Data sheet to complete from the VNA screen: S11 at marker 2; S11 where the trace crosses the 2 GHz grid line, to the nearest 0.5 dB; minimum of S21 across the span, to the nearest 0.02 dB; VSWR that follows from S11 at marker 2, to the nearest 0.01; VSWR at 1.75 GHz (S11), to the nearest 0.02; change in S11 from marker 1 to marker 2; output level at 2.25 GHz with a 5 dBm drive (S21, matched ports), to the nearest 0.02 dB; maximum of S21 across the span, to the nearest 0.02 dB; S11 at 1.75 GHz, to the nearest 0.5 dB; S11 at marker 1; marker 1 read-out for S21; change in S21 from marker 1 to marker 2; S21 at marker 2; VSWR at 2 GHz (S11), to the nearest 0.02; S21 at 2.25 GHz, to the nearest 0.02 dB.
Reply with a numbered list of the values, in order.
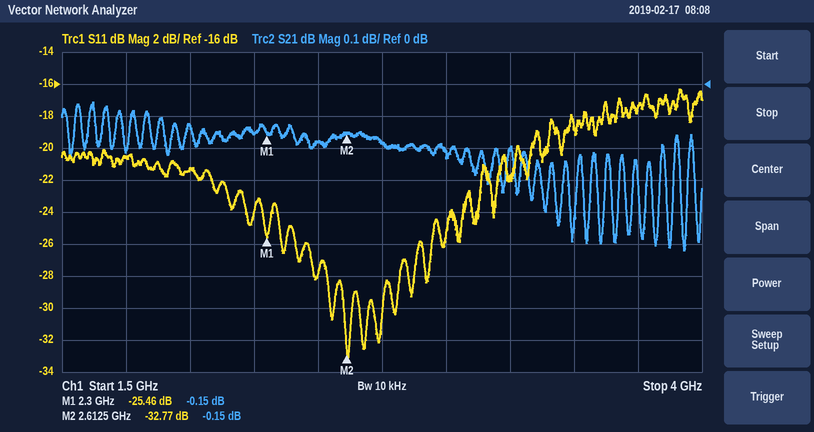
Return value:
1. -32.77 dB
2. -21.5 dB
3. -0.52 dB
4. 1.05
5. 1.20
6. -7.31 dB
7. 4.84 dBm
8. -0.06 dB
9. -20.5 dB
10. -25.46 dB
11. -0.15 dB
12. 0.00 dB
13. -0.15 dB
14. 1.18
15. -0.16 dB
